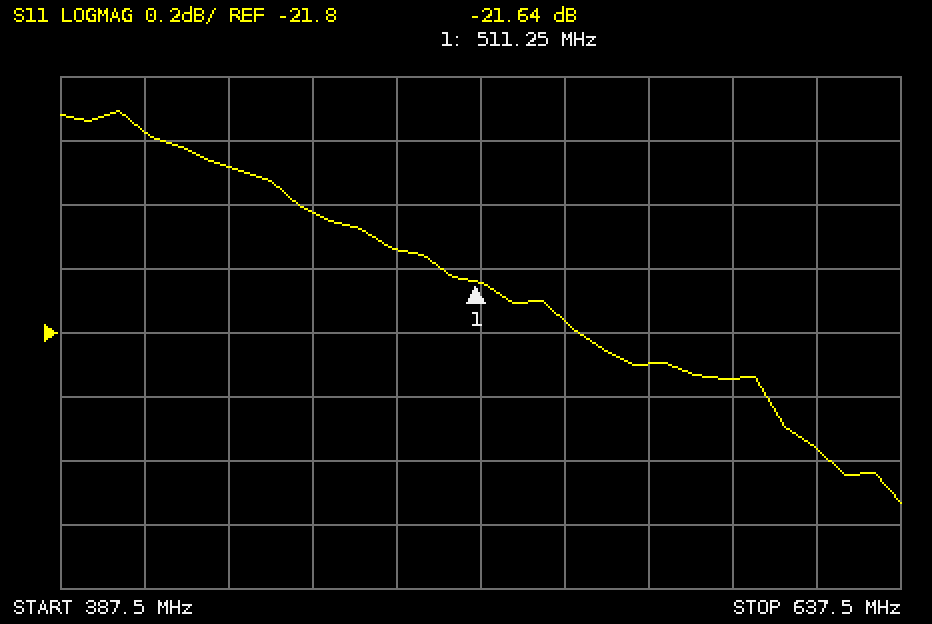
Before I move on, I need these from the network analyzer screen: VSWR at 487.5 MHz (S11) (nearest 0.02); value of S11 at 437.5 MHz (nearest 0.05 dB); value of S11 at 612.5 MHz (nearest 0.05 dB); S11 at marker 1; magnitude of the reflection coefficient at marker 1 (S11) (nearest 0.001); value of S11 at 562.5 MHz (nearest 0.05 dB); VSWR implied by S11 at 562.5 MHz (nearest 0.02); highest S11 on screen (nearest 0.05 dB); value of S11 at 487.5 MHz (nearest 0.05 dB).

1.18
-21.30 dB
-22.15 dB
-21.64 dB
0.083
-21.90 dB
1.18
-21.10 dB
-21.55 dB
